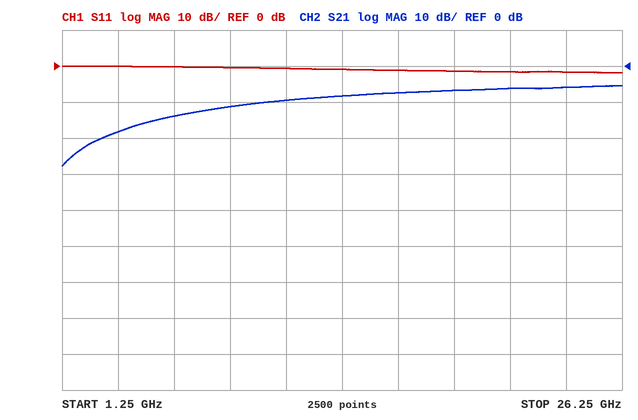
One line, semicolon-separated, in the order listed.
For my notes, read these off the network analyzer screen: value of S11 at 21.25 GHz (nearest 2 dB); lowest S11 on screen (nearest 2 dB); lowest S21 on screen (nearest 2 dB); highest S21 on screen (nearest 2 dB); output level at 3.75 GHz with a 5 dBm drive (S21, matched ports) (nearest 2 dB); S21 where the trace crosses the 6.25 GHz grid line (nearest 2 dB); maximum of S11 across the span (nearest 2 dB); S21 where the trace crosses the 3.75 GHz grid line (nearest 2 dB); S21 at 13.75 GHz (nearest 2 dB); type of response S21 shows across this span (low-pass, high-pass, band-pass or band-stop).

-2 dB; -2 dB; -28 dB; -6 dB; -14 dBm; -14 dB; 0 dB; -18 dB; -8 dB; high-pass
